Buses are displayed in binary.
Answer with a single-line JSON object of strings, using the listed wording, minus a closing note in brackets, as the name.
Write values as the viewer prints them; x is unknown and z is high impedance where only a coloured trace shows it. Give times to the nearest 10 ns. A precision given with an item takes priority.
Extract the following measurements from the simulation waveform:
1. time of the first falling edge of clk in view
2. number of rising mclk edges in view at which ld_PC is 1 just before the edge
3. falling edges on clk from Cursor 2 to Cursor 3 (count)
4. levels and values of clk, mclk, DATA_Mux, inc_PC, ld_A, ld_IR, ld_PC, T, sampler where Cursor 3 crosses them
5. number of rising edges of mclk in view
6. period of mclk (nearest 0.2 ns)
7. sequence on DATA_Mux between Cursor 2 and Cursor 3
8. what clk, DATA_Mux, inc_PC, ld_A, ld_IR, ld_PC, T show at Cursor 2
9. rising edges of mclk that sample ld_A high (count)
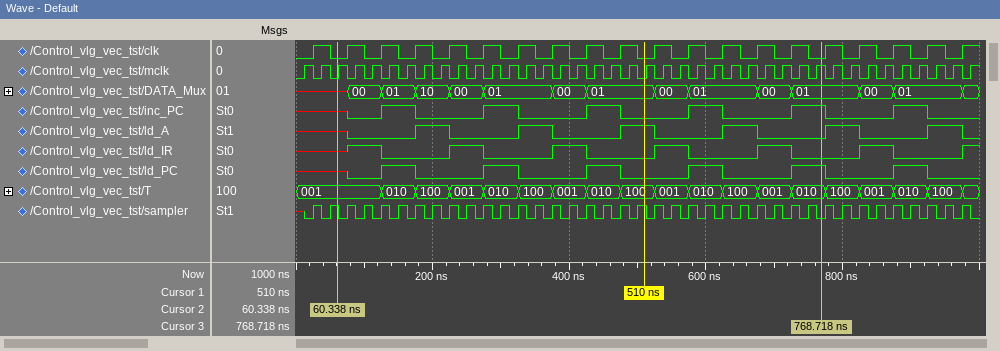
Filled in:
{"time of the first falling edge of clk in view": "50 ns", "number of rising mclk edges in view at which ld_PC is 1 just before the edge": "12", "falling edges on clk from Cursor 2 to Cursor 3": "14", "levels and values of clk, mclk, DATA_Mux, inc_PC, ld_A, ld_IR, ld_PC, T, sampler where Cursor 3 crosses them": "clk=0, mclk=1, DATA_Mux=01, inc_PC=1, ld_A=0, ld_IR=0, ld_PC=1, T=010, sampler=0", "number of rising edges of mclk in view": "40", "period of mclk": "25 ns", "sequence on DATA_Mux between Cursor 2 and Cursor 3": "x, 00, 01, 10, 00, 01, 00, 01, 00, 01, 00, 01", "what clk, DATA_Mux, inc_PC, ld_A, ld_IR, ld_PC, T show at Cursor 2": "clk=0, DATA_Mux=x, inc_PC=x, ld_A=x, ld_IR=x, ld_PC=x, T=001", "rising edges of mclk that sample ld_A high": "12"}
